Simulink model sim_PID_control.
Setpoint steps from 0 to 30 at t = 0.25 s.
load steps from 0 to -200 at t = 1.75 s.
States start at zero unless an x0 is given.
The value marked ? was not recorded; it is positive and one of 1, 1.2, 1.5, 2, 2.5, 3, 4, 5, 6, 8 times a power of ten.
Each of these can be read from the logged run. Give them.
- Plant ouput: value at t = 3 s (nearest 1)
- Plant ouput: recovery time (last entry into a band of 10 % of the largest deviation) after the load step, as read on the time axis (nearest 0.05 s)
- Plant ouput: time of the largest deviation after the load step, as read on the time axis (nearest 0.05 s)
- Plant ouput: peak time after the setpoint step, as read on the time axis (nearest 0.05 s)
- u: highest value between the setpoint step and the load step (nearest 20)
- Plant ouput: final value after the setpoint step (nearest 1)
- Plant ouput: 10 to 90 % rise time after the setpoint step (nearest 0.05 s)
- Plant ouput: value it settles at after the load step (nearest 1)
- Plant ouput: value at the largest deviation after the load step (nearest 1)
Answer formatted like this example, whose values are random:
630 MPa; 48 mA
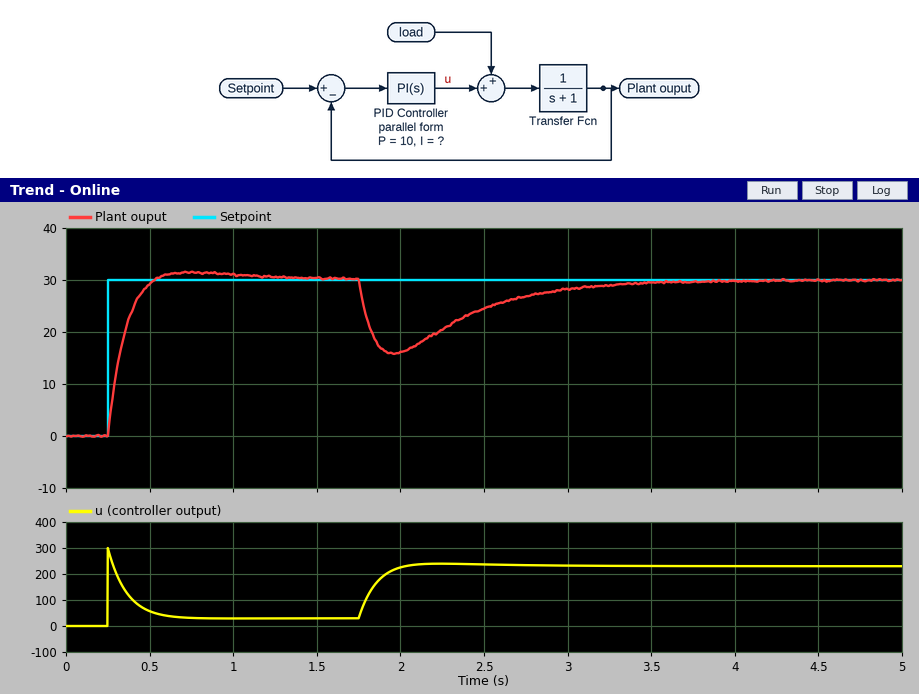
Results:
28; 3.10 s; 1.95 s; 0.75 s; 300; 30; 0.20 s; 30; 16
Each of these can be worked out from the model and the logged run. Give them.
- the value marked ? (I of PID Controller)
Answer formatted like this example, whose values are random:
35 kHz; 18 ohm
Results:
20
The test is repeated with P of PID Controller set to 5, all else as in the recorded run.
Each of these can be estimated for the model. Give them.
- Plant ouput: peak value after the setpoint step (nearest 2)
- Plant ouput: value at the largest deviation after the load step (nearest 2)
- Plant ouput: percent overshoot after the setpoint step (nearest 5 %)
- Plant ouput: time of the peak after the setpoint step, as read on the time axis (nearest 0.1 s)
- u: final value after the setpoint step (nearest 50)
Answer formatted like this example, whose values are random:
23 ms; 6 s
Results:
34; 8; 15 %; 0.8 s; 50
